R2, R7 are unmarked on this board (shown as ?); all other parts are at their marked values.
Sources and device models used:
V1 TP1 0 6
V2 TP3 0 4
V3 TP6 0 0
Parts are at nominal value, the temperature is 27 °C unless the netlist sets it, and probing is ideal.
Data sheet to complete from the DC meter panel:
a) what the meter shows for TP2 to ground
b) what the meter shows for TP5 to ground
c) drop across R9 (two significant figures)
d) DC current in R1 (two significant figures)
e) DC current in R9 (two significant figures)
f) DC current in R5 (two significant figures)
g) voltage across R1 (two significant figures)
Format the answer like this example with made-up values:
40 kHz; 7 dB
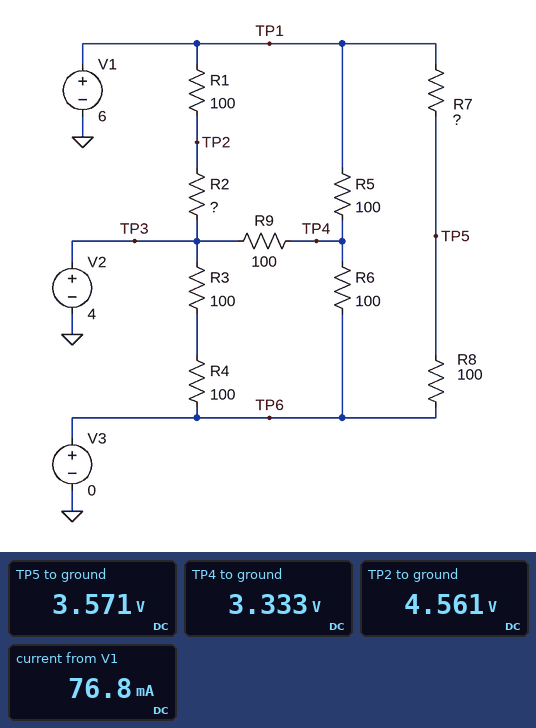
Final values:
4.561 V; 3.571 V; 670 mV; 14 mA; 6.7 mA; 27 mA; 1.4 V
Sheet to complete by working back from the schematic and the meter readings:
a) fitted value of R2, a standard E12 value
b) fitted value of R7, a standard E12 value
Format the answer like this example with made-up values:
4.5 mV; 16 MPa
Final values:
39 Ω; 68 Ω
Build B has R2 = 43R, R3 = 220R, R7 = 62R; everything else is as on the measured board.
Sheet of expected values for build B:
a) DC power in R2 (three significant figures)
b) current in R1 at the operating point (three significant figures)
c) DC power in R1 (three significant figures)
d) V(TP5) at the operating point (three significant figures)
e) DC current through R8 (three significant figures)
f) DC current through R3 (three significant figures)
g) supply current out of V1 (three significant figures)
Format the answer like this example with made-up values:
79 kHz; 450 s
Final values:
8.41 mW; 14.0 mA; 19.6 mW; 3.70 V; 37.0 mA; 12.5 mA; 77.7 mA
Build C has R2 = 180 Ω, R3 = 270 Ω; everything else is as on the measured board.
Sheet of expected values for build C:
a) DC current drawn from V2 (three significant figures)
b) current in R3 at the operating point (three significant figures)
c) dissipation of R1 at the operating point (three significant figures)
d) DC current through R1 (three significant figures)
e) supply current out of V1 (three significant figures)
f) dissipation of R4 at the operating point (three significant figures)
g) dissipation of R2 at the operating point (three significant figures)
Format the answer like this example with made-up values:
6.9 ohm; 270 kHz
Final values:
10.3 mA; 10.8 mA; 5.10 mW; 7.14 mA; 69.5 mA; 11.7 mW; 9.18 mW
